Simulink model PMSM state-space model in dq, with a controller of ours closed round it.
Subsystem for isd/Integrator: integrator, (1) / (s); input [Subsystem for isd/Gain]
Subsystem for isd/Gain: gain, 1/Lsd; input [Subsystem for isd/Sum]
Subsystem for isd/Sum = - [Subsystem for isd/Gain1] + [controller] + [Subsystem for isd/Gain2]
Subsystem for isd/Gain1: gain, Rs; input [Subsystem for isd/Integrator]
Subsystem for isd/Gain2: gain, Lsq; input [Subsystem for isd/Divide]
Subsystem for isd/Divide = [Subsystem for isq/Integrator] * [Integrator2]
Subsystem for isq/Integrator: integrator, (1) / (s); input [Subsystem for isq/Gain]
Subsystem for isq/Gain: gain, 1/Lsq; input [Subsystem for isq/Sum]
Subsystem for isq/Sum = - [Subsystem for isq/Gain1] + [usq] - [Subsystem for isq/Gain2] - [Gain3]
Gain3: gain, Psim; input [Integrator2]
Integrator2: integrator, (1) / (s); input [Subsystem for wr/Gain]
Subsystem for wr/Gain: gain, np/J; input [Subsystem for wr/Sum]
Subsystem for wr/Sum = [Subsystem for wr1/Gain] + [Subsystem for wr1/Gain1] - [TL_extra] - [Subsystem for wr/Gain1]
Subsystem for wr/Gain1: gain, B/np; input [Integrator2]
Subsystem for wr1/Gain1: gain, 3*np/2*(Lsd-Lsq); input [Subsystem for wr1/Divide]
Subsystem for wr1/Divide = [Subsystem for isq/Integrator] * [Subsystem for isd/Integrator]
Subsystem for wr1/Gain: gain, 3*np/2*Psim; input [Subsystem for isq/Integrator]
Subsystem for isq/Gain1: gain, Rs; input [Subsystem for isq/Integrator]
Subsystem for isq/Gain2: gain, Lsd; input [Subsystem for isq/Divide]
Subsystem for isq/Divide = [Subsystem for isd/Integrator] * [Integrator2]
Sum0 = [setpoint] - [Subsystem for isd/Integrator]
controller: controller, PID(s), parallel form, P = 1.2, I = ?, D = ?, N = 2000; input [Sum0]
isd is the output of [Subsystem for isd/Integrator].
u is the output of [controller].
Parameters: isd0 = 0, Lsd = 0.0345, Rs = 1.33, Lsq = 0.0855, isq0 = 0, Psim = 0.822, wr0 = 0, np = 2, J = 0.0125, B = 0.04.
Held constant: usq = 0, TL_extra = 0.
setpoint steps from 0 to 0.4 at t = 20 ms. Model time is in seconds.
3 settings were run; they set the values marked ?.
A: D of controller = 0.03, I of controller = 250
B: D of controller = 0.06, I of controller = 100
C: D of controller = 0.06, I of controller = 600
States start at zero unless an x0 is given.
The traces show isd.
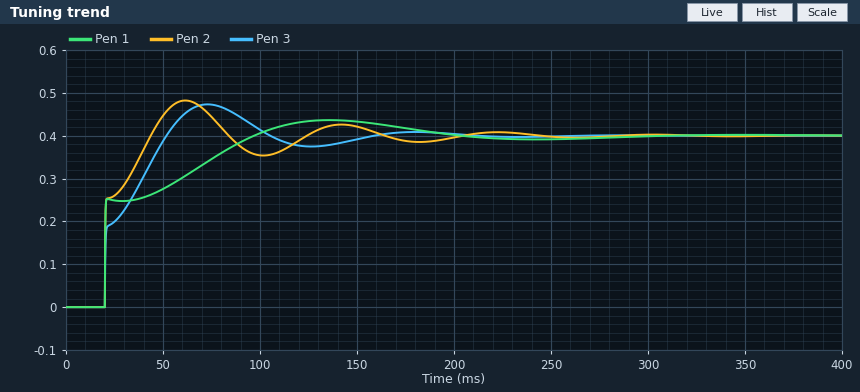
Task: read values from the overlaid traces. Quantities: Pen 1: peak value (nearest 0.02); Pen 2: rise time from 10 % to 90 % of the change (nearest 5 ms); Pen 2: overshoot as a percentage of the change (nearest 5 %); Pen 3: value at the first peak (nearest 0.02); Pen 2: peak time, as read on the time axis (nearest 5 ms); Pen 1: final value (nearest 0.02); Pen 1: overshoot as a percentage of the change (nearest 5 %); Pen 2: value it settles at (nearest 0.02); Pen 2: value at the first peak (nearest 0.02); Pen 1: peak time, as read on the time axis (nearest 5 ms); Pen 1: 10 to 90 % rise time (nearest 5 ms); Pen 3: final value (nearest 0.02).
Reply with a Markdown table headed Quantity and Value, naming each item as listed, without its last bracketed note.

| Quantity | Value |
|---|---|
| Pen 1: peak value | 0.44 |
| Pen 2: rise time from 10 % to 90 % of the change | 20 ms |
| Pen 2: overshoot as a percentage of the change | 20 % |
| Pen 3: value at the first peak | 0.48 |
| Pen 2: peak time, as read on the time axis | 60 ms |
| Pen 1: final value | 0.40 |
| Pen 1: overshoot as a percentage of the change | 10 % |
| Pen 2: value it settles at | 0.40 |
| Pen 2: value at the first peak | 0.48 |
| Pen 1: peak time, as read on the time axis | 135 ms |
| Pen 1: 10 to 90 % rise time | 60 ms |
| Pen 3: final value | 0.40 |
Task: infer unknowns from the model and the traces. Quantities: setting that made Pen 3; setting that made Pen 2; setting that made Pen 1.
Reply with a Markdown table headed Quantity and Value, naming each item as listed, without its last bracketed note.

| Quantity | Value |
|---|---|
| setting that made Pen 3 | A |
| setting that made Pen 2 | C |
| setting that made Pen 1 | B |
